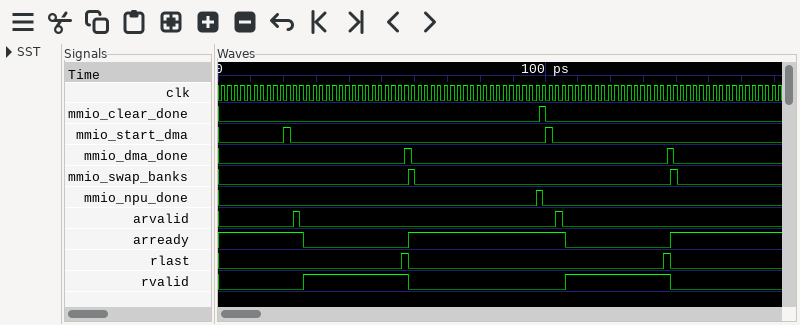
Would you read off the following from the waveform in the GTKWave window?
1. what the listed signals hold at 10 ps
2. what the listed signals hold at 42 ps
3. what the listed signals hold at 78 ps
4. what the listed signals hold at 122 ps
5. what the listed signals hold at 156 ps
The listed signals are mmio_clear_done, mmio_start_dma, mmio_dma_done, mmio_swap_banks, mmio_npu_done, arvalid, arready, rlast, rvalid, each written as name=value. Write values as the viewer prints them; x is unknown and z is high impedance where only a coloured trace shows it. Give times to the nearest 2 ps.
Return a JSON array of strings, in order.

["mmio_clear_done=0, mmio_start_dma=0, mmio_dma_done=0, mmio_swap_banks=0, mmio_npu_done=0, arvalid=0, arready=1, rlast=0, rvalid=0", "mmio_clear_done=0, mmio_start_dma=0, mmio_dma_done=0, mmio_swap_banks=0, mmio_npu_done=0, arvalid=0, arready=0, rlast=0, rvalid=1", "mmio_clear_done=0, mmio_start_dma=0, mmio_dma_done=0, mmio_swap_banks=0, mmio_npu_done=0, arvalid=0, arready=1, rlast=0, rvalid=0", "mmio_clear_done=0, mmio_start_dma=0, mmio_dma_done=0, mmio_swap_banks=0, mmio_npu_done=0, arvalid=0, arready=0, rlast=0, rvalid=1", "mmio_clear_done=0, mmio_start_dma=0, mmio_dma_done=0, mmio_swap_banks=0, mmio_npu_done=0, arvalid=0, arready=1, rlast=0, rvalid=0"]
